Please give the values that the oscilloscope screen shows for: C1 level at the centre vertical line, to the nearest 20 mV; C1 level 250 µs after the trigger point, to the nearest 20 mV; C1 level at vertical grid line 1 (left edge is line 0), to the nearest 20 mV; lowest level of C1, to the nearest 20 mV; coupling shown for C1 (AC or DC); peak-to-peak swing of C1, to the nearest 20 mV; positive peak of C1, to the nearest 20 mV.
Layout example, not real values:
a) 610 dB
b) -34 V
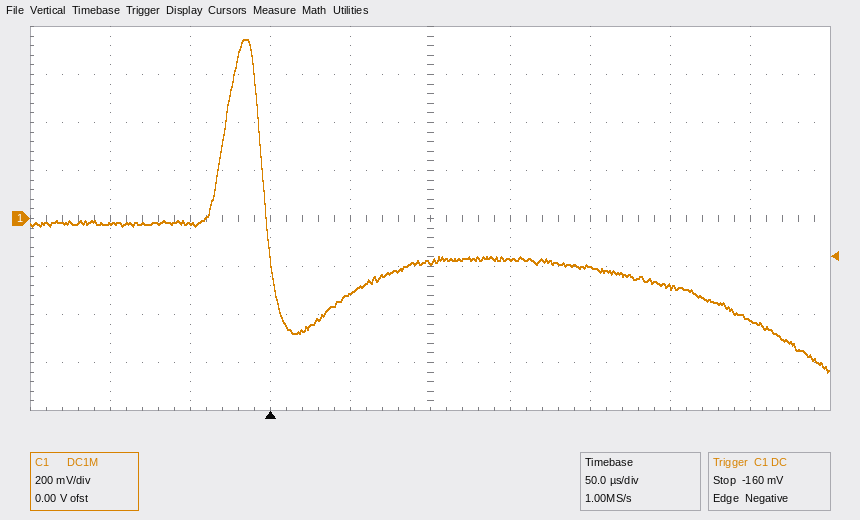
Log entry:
a) -180 mV
b) -280 mV
c) -20 mV
d) -640 mV
e) DC
f) 1.38 V
g) 740 mV
